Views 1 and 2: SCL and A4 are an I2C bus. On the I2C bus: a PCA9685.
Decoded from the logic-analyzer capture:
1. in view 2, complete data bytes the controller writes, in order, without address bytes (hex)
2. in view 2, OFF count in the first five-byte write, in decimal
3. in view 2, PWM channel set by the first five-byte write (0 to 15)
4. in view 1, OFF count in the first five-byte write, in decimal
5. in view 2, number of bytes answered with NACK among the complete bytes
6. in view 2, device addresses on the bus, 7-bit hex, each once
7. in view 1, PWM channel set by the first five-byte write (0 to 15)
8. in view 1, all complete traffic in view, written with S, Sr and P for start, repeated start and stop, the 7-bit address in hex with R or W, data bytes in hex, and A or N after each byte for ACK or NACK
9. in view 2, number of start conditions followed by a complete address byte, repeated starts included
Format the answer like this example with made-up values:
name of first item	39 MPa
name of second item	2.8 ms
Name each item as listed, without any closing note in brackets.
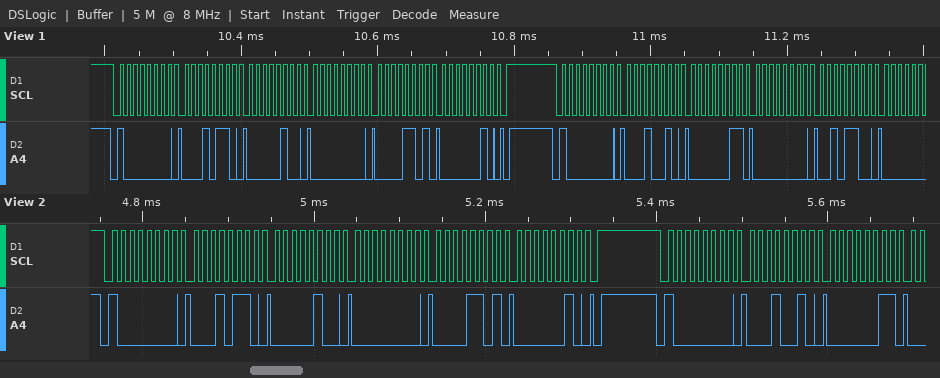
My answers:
in view 2, complete data bytes the controller writes, in order, without address bytes	16 04 00 0D 02 12 03
in view 2, OFF count in the first five-byte write, in decimal	525
in view 2, PWM channel set by the first five-byte write	4
in view 1, OFF count in the first five-byte write, in decimal	525
in view 2, number of bytes answered with NACK among the complete bytes	0
in view 2, device addresses on the bus, 7-bit hex, each once	0x40
in view 1, PWM channel set by the first five-byte write	4
in view 1, all complete traffic in view, written with S, Sr and P for start, repeated start and stop, the 7-bit address in hex with R or W, data bytes in hex, and A or N after each byte for ACK or NACK	S 40W A 16 A 04 A 00 A 0D A 02 A P S 40W A 12 A 03 A 00 A 2C A
in view 2, number of start conditions followed by a complete address byte, repeated starts included	2
